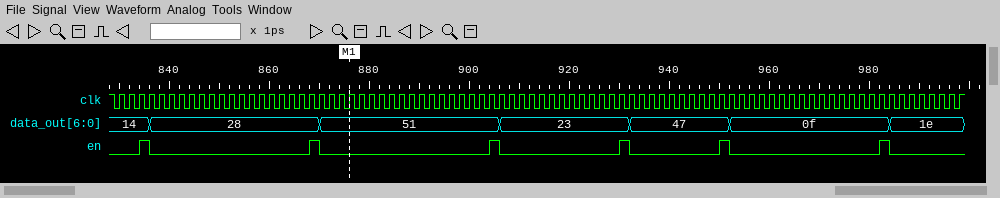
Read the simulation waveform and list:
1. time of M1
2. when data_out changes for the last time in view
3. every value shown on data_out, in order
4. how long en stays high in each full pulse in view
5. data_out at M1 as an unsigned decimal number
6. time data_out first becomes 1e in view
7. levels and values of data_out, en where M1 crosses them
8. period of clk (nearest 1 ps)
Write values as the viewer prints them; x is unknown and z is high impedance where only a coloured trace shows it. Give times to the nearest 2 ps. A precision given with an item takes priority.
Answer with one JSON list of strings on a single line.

["876 ps", "984 ps", "14, 28, 51, 23, 47, 0f, 1e", "2 ps, 2 ps, 2 ps, 2 ps, 2 ps, 2 ps", "81", "984 ps", "data_out=51, en=0", "2 ps"]
